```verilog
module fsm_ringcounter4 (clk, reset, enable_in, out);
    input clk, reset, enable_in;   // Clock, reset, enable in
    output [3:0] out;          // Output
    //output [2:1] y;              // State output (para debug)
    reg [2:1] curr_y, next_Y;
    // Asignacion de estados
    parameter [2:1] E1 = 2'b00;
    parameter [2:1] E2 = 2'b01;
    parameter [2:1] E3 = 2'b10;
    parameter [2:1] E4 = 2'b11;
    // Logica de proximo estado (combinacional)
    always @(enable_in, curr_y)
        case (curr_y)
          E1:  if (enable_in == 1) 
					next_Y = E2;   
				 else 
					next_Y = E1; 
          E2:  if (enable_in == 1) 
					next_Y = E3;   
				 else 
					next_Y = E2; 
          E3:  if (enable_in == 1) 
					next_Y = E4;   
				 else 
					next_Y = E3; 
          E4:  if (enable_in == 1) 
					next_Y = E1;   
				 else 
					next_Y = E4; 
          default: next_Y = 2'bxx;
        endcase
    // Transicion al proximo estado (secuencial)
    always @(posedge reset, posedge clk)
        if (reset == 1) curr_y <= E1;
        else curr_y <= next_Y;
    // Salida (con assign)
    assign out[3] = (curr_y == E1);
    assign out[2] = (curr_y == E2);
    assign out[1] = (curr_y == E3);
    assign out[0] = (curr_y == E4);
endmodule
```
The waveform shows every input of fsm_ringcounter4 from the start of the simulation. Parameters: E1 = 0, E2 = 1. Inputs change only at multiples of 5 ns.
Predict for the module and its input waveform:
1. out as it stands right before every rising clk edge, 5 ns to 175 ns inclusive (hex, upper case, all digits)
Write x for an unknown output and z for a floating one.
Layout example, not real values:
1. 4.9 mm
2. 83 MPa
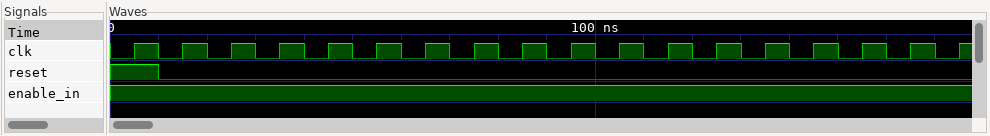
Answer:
1. 8, 8, 4, 2, 1, 8, 4, 2, 1, 8, 4, 2, 1, 8, 4, 2, 1, 8
